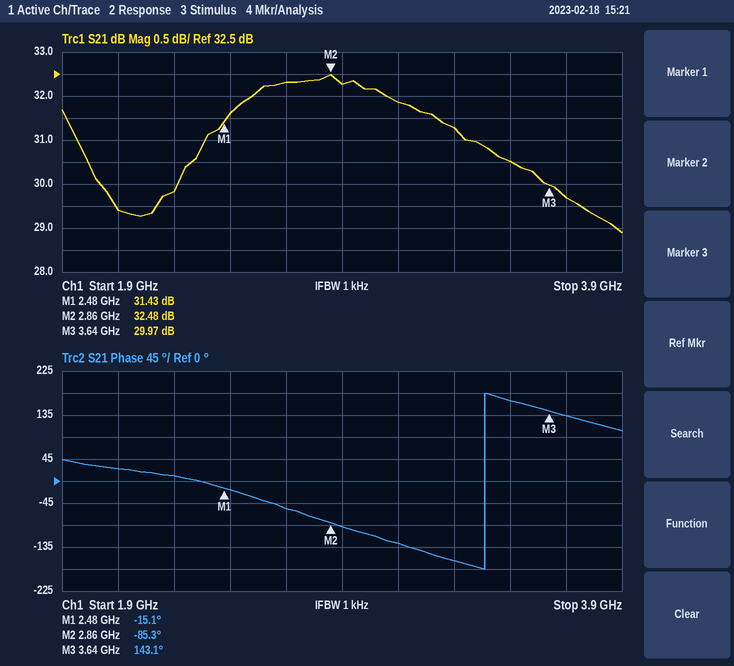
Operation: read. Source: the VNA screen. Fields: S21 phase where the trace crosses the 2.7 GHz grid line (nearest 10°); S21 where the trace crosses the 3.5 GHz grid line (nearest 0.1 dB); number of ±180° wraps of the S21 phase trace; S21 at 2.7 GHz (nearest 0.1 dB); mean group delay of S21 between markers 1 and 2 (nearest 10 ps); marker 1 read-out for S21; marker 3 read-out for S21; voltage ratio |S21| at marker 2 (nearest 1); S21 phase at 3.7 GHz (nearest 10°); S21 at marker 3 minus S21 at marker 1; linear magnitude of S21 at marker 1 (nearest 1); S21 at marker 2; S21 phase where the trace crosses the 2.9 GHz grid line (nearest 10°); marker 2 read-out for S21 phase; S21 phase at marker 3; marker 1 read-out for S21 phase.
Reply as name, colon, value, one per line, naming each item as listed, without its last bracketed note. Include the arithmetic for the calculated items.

S21 phase where the trace crosses the 2.7 GHz grid line: -60°
S21 where the trace crosses the 3.5 GHz grid line: 30.5 dB
number of ±180° wraps of the S21 phase trace: 1
S21 at 2.7 GHz: 32.3 dB
mean group delay of S21 between markers 1 and 2: −(-85.3° − (-15.1°))/(360° × 380 MHz) ≈ 513 ps, so 510 ps to the nearest 10 ps
marker 1 read-out for S21: 31.43 dB
marker 3 read-out for S21: 29.97 dB
voltage ratio |S21| at marker 2: 10^(32.48/20) ≈ 42
S21 phase at 3.7 GHz: 130°
S21 at marker 3 minus S21 at marker 1: 29.97 − (31.43) = -1.46 dB
linear magnitude of S21 at marker 1: 10^(31.43/20) ≈ 37
S21 at marker 2: 32.48 dB
S21 phase where the trace crosses the 2.9 GHz grid line: -90°
marker 2 read-out for S21 phase: -85.3°
S21 phase at marker 3: 143.1°
marker 1 read-out for S21 phase: -15.1°
